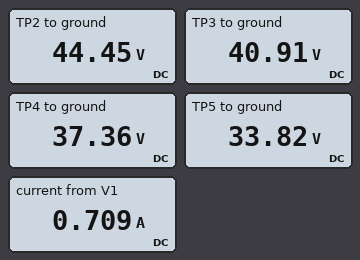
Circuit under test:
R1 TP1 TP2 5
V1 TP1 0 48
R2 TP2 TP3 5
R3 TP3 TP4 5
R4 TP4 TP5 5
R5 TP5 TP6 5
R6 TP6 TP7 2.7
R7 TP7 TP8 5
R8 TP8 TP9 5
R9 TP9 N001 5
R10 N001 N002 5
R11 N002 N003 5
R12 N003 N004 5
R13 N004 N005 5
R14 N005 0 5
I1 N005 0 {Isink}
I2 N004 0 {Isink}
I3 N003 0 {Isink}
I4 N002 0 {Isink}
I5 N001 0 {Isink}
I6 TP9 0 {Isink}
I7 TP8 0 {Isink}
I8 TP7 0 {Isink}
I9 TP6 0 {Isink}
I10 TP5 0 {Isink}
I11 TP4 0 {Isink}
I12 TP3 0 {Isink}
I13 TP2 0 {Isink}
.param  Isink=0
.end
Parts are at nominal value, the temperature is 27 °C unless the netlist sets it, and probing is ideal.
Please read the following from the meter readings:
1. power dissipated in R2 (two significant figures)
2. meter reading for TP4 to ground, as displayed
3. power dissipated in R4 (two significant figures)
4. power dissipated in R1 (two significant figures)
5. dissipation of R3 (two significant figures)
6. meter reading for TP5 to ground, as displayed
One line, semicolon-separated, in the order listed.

2.5 W; 37.36 V; 2.5 W; 2.5 W; 2.5 W; 33.82 V
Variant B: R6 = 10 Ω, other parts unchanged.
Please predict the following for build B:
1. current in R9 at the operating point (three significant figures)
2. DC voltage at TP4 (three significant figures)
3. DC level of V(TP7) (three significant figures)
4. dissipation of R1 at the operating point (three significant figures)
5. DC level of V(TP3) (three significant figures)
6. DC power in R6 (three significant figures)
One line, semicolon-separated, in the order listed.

640 mA; 38.4 V; 25.6 V; 2.05 W; 41.6 V; 4.10 W
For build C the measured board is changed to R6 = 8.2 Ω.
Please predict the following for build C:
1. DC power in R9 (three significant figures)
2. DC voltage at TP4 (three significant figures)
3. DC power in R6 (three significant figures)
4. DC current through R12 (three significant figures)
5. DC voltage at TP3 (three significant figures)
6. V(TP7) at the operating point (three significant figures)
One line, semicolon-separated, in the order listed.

2.15 W; 38.2 V; 3.53 W; 656 mA; 41.4 V; 26.2 V
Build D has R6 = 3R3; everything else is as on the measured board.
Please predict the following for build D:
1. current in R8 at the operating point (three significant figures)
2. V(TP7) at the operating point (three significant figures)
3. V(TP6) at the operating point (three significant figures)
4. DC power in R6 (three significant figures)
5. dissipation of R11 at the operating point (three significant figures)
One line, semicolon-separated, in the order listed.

703 mA; 28.1 V; 30.4 V; 1.63 W; 2.47 W
